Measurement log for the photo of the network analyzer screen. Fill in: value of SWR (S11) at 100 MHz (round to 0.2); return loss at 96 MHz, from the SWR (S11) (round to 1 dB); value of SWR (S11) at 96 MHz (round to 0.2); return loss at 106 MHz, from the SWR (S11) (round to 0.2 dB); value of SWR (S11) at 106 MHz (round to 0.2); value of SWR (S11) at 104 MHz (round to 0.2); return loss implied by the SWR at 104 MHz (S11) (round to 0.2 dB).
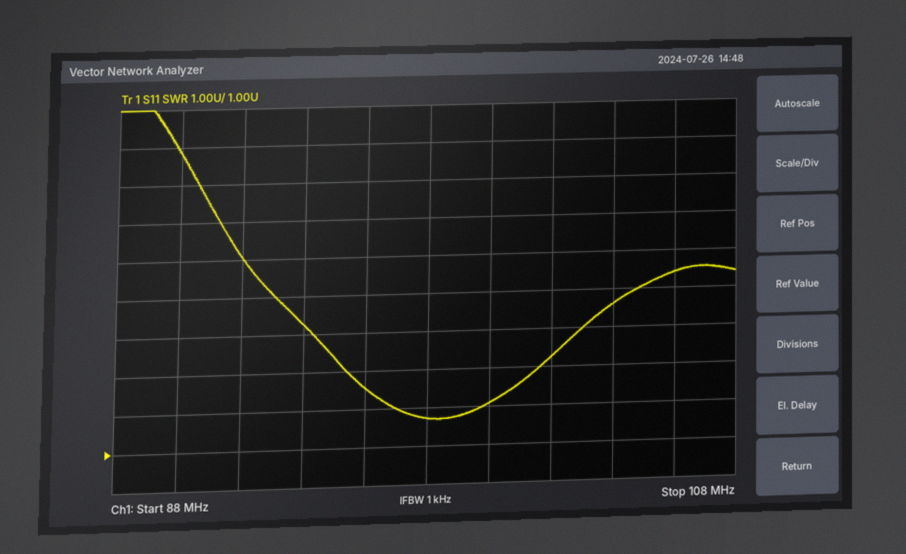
2.0
7 dB
2.6
3.2 dB
5.4
4.6
3.8 dB
